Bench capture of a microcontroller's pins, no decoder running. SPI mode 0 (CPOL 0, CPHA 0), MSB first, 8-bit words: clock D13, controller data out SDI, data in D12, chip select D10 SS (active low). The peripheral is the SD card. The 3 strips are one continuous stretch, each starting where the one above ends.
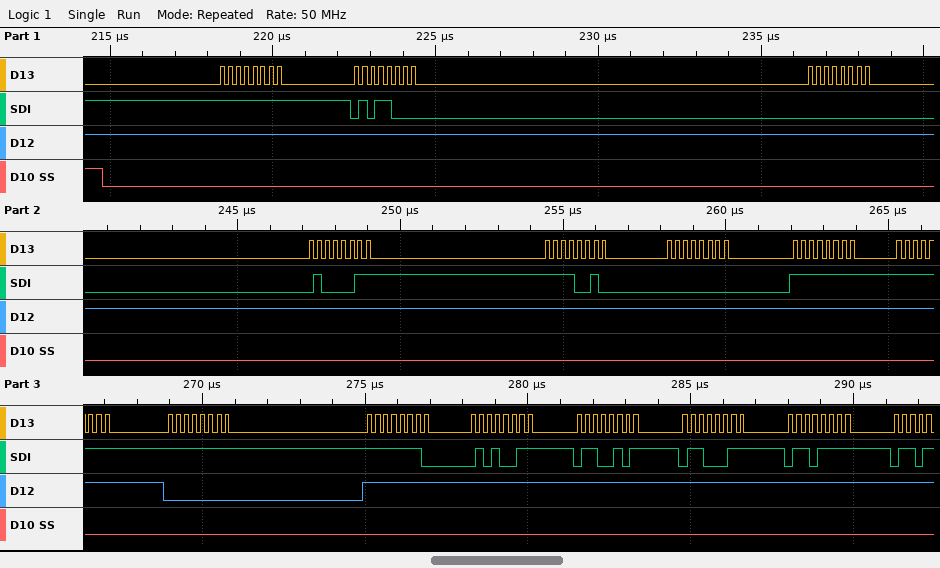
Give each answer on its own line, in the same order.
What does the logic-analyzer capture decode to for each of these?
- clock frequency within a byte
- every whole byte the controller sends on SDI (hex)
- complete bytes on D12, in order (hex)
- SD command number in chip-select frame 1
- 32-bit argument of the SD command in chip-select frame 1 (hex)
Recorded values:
4 MHz
FF 58 00 43 F2 00 FF FF FF FE 53 65 63 6F
FF FF FF FF FF FF FF FF 00 FF FF FF FF FF
CMD24
0x0043F200
